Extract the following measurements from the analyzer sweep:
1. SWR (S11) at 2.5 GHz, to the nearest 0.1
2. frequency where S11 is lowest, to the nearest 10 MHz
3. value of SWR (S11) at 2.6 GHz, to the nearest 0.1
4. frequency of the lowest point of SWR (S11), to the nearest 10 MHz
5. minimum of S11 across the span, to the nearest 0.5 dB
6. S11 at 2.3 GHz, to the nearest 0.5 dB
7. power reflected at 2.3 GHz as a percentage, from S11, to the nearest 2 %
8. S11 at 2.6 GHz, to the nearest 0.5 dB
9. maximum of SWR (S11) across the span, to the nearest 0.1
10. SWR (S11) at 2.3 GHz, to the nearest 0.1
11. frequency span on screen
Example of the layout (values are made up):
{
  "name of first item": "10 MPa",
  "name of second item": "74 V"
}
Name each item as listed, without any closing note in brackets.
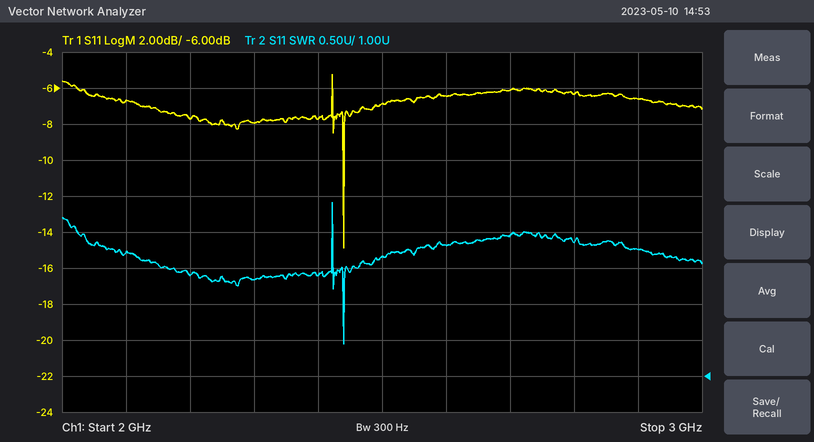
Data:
{
  "SWR (S11) at 2.5 GHz, to the nearest 0.1": "2.7",
  "frequency where S11 is lowest, to the nearest 10 MHz": "2.44 GHz",
  "value of SWR (S11) at 2.6 GHz, to the nearest 0.1": "2.8",
  "frequency of the lowest point of SWR (S11), to the nearest 10 MHz": "2.44 GHz",
  "minimum of S11 across the span, to the nearest 0.5 dB": "-15.0 dB",
  "S11 at 2.3 GHz, to the nearest 0.5 dB": "-8.0 dB",
  "power reflected at 2.3 GHz as a percentage, from S11, to the nearest 2 %": "16 %",
  "S11 at 2.6 GHz, to the nearest 0.5 dB": "-6.5 dB",
  "maximum of SWR (S11) across the span, to the nearest 0.1": "3.4",
  "SWR (S11) at 2.3 GHz, to the nearest 0.1": "2.3",
  "frequency span on screen": "1 GHz"
}
